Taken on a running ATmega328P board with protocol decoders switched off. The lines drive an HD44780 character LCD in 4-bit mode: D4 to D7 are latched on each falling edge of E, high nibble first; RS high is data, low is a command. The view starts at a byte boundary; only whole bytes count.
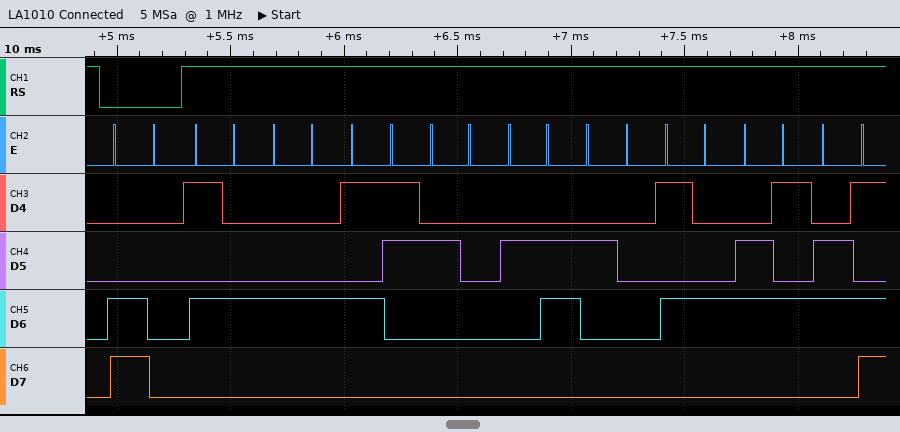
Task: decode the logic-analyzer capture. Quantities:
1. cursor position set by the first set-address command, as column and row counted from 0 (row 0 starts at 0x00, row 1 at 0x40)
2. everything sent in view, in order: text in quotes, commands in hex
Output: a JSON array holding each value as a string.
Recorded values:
["column 0, row 1", "0xC0 \"TDS & Tem\""]
